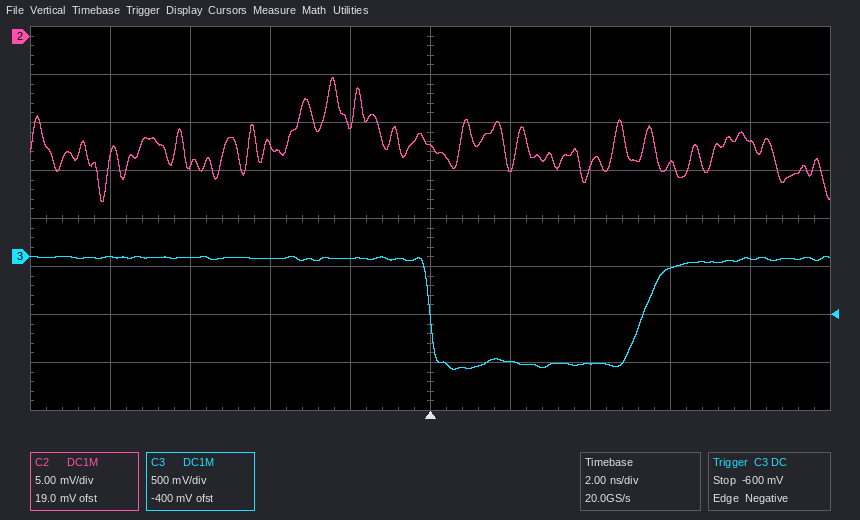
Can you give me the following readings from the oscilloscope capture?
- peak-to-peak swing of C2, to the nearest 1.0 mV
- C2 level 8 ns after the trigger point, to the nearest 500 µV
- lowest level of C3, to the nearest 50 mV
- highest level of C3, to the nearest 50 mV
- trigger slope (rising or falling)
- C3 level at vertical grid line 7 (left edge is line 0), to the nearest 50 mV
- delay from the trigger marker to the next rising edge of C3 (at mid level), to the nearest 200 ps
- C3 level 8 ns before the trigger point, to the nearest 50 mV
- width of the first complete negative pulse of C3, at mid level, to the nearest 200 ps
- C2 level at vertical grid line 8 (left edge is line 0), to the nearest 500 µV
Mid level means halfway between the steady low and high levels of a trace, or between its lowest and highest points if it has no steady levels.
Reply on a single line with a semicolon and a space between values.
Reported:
13.0 mV; -11.0 mV; -1.15 V; 0 mV; falling; -1.10 V; 5.4 ns; 0 mV; 5.4 ns; -13.5 mV
